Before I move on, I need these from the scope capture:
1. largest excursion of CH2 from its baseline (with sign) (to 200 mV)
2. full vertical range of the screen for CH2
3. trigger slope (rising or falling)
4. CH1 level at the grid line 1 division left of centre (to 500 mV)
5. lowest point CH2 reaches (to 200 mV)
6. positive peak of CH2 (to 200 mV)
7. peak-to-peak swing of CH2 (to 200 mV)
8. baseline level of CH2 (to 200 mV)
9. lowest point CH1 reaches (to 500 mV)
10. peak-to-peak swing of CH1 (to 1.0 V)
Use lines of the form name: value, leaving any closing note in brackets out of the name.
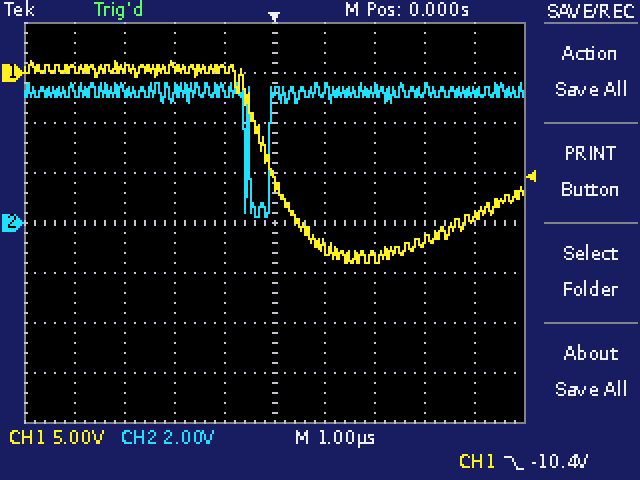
largest excursion of CH2 from its baseline (with sign): -5.0 V
full vertical range of the screen for CH2: 16 V
trigger slope: falling
CH1 level at the grid line 1 division left of centre: 500 mV
lowest point CH2 reaches: 200 mV
positive peak of CH2: 5.6 V
peak-to-peak swing of CH2: 5.4 V
baseline level of CH2: 5.2 V
lowest point CH1 reaches: -19.0 V
peak-to-peak swing of CH1: 20.0 V
